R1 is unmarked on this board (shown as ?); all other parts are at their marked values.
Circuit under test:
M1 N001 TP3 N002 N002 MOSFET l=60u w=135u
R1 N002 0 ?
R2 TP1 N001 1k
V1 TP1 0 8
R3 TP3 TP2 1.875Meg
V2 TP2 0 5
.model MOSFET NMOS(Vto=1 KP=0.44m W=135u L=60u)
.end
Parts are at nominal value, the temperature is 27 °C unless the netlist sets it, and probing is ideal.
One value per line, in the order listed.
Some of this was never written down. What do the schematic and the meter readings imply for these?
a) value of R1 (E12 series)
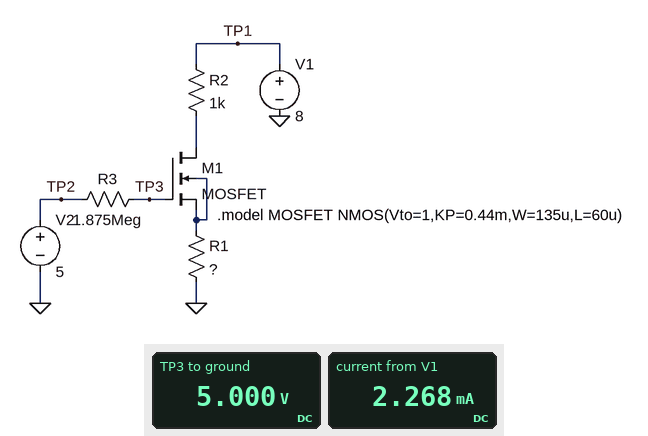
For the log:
820 Ω
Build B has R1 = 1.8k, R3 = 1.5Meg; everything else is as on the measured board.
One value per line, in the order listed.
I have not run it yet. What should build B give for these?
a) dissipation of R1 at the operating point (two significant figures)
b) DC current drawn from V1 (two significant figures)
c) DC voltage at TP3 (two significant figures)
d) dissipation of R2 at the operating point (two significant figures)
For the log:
3.1 mW
1.3 mA
5.0 V
1.7 mW
